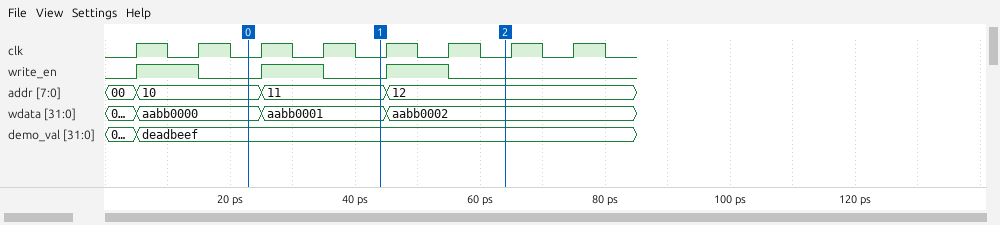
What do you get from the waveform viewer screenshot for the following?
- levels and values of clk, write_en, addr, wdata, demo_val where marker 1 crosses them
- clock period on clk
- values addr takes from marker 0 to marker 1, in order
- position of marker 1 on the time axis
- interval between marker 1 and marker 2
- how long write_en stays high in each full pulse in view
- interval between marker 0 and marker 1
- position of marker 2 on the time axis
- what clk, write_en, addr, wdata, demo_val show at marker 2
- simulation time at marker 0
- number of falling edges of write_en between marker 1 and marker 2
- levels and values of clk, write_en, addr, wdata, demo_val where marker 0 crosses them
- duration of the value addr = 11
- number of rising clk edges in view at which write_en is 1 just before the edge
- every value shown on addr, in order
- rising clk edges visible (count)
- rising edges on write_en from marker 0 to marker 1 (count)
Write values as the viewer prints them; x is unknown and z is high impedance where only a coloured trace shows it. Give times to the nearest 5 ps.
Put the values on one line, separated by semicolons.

clk=0, write_en=0, addr=11, wdata=aabb0001, demo_val=deadbeef; 10 ps; 10, 11; 45 ps; 20 ps; 10 ps, 10 ps, 10 ps; 20 ps; 65 ps; clk=0, write_en=0, addr=12, wdata=aabb0002, demo_val=deadbeef; 25 ps; 1; clk=0, write_en=0, addr=10, wdata=aabb0000, demo_val=deadbeef; 20 ps; 3; 00, 10, 11, 12; 8; 1
